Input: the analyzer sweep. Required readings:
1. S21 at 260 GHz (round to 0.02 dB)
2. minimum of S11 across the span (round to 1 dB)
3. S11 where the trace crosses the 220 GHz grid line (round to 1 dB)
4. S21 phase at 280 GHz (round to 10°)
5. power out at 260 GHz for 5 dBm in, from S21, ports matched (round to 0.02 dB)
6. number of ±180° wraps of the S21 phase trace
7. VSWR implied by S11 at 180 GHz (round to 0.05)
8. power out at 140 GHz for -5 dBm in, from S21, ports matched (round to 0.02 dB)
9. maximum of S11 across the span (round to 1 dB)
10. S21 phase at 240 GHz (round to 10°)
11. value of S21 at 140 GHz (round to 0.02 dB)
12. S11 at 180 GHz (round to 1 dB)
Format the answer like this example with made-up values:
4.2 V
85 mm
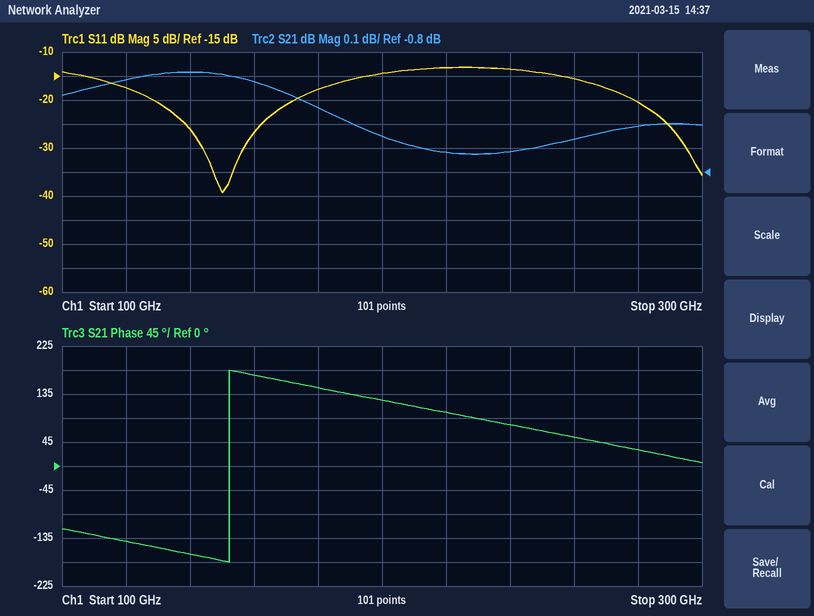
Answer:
-0.66 dB
-39 dB
-13 dB
30°
4.34 dBm
1
1.30
-5.38 dBm
-13 dB
80°
-0.38 dB
-18 dB
